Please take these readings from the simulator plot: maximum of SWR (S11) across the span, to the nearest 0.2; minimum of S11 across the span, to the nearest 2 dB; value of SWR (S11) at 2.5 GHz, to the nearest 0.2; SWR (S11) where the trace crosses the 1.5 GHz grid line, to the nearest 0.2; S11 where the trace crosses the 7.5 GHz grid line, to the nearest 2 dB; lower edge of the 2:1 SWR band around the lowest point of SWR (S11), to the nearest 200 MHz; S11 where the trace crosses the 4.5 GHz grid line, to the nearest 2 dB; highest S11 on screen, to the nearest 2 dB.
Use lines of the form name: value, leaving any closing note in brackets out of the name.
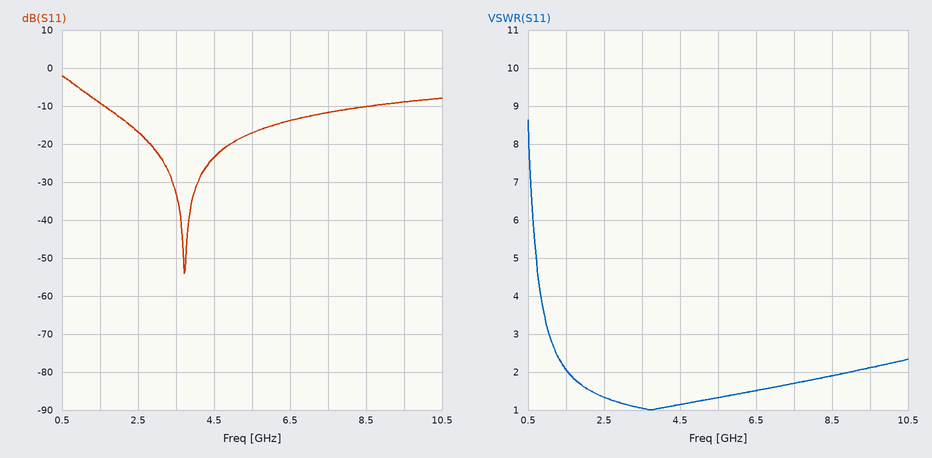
maximum of SWR (S11) across the span, to the nearest 0.2: 8.6
minimum of S11 across the span, to the nearest 2 dB: -54 dB
value of SWR (S11) at 2.5 GHz, to the nearest 0.2: 1.4
SWR (S11) where the trace crosses the 1.5 GHz grid line, to the nearest 0.2: 2.0
S11 where the trace crosses the 7.5 GHz grid line, to the nearest 2 dB: -12 dB
lower edge of the 2:1 SWR band around the lowest point of SWR (S11), to the nearest 200 MHz: 1.6 GHz
S11 where the trace crosses the 4.5 GHz grid line, to the nearest 2 dB: -24 dB
highest S11 on screen, to the nearest 2 dB: -2 dB
